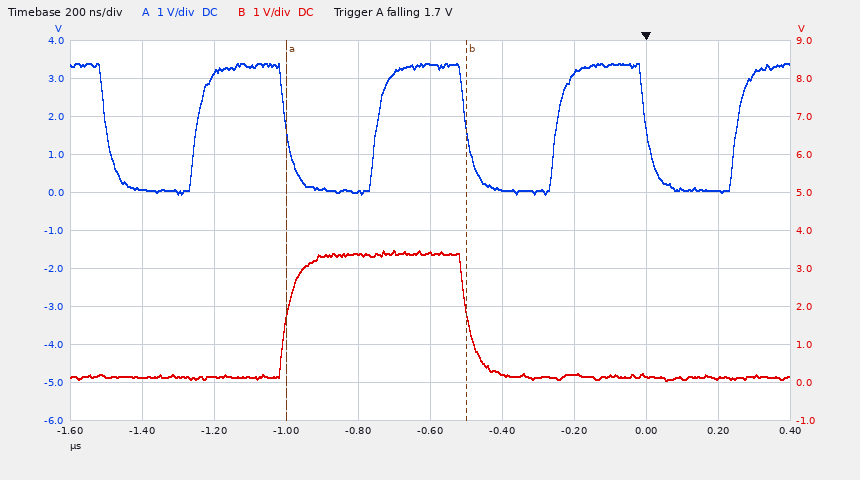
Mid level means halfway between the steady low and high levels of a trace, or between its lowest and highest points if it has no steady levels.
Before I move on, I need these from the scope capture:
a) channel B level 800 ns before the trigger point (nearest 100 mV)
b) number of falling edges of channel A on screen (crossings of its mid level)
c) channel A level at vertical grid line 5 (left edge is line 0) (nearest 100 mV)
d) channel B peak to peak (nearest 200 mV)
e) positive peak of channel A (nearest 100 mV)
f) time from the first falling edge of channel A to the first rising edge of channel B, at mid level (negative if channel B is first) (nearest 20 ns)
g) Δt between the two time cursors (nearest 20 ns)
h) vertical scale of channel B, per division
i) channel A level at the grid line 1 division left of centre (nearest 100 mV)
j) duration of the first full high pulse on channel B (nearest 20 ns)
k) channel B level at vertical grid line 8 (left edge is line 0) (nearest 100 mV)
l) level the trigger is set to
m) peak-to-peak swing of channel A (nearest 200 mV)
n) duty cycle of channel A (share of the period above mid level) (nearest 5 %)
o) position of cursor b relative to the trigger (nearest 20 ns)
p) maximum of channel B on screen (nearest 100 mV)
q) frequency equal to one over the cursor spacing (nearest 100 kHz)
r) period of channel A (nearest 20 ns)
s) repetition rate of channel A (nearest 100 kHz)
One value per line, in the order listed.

3.4 V
4
3.4 V
3.4 V
3.4 V
+500 ns
500 ns
1 V
0.0 V
500 ns
200 mV
1.7 V
3.4 V
50 %
-500 ns
3.5 V
2.0 MHz
500 ns
2.0 MHz
